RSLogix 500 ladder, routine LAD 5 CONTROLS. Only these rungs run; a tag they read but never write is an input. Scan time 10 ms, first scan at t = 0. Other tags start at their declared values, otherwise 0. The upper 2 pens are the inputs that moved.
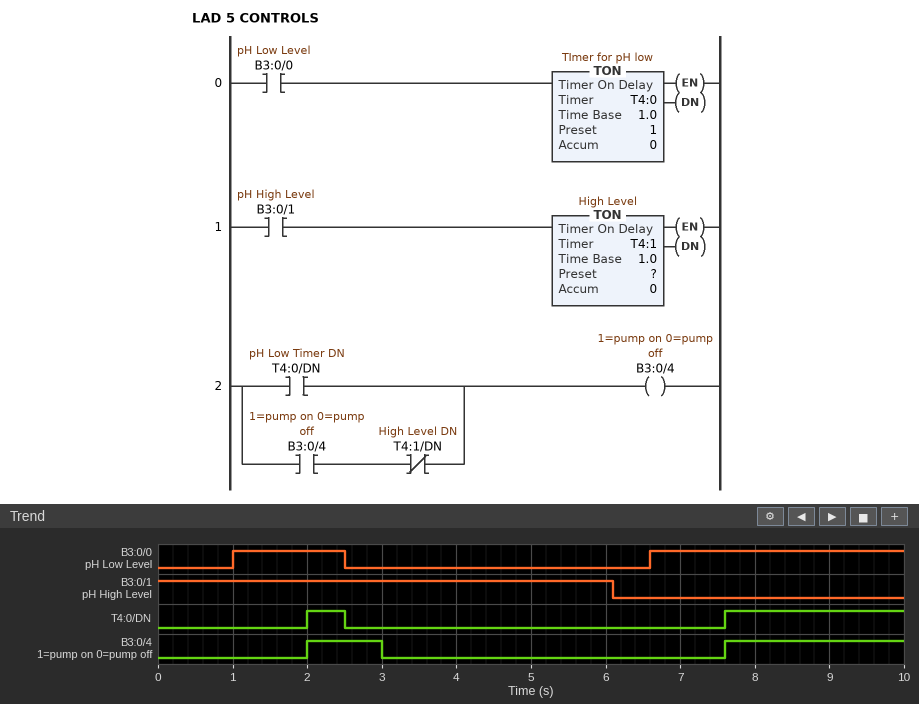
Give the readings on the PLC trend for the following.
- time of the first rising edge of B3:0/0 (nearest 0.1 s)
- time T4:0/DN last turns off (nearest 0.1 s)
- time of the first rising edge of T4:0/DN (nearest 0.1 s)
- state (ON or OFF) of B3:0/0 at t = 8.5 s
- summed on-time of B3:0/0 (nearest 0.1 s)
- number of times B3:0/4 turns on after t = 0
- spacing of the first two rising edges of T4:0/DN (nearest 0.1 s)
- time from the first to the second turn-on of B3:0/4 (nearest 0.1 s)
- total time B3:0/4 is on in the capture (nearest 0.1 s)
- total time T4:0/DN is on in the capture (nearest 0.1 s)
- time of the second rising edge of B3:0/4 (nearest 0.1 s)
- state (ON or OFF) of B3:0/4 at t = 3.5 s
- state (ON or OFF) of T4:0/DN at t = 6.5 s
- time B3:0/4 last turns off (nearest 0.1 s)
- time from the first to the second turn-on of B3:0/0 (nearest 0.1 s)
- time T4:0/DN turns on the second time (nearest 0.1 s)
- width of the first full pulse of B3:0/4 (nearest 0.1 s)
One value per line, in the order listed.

1.0 s
2.5 s
2.0 s
ON
4.9 s
2
5.6 s
5.6 s
3.4 s
2.9 s
7.6 s
OFF
OFF
3.0 s
5.6 s
7.6 s
1.0 s
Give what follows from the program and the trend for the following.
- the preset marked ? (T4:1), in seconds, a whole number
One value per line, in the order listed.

3 s
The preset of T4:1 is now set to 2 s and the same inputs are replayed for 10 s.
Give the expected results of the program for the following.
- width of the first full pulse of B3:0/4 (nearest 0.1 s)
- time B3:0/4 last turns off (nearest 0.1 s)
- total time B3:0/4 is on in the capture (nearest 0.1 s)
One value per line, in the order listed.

0.5 s
2.5 s
2.9 s
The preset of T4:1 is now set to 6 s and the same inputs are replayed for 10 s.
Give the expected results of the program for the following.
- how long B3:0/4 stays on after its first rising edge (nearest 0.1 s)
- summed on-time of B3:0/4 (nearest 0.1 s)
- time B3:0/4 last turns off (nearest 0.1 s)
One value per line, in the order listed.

4.0 s
6.4 s
6.0 s
